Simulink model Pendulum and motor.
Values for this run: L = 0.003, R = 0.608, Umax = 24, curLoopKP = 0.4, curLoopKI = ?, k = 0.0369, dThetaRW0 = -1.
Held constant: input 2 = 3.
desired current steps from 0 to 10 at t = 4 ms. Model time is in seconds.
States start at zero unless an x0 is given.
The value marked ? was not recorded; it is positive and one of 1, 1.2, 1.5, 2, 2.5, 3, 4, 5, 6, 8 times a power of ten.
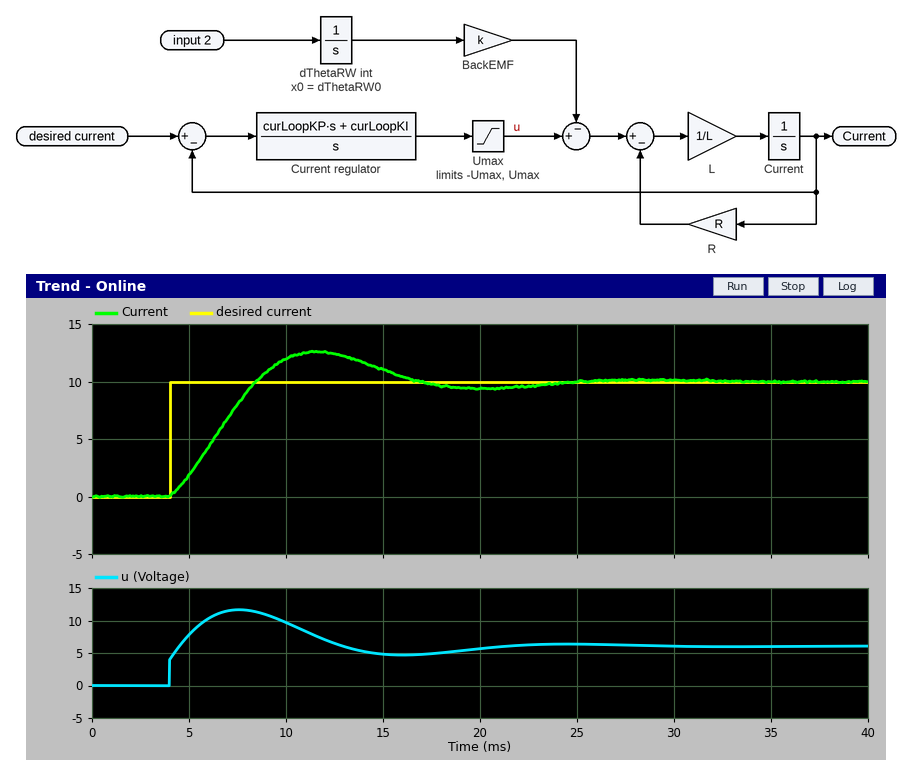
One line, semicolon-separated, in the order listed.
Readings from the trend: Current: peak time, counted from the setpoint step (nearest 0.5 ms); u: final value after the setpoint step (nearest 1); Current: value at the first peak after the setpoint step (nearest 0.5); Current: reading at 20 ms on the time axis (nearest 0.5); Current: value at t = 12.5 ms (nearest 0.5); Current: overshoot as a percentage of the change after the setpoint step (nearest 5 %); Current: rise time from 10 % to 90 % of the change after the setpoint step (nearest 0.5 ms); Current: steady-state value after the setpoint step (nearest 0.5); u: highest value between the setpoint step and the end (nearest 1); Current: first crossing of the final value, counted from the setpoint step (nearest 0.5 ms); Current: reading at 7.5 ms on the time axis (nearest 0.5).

7.5 ms; 6; 12.5; 9.5; 12.5; 25 %; 3.5 ms; 10.0; 12; 4.5 ms; 8.0
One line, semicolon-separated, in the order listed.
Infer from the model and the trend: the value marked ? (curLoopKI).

500
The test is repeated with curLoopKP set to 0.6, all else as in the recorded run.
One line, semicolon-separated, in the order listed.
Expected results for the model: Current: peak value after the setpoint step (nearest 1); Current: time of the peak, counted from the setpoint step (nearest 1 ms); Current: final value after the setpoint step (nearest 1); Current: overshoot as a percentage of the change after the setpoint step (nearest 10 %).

12; 7 ms; 10; 20 %
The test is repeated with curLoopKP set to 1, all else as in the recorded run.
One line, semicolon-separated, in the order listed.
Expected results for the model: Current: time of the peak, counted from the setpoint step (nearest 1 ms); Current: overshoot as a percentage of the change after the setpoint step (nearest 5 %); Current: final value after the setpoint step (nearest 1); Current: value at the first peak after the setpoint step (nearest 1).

7 ms; 10 %; 10; 11
